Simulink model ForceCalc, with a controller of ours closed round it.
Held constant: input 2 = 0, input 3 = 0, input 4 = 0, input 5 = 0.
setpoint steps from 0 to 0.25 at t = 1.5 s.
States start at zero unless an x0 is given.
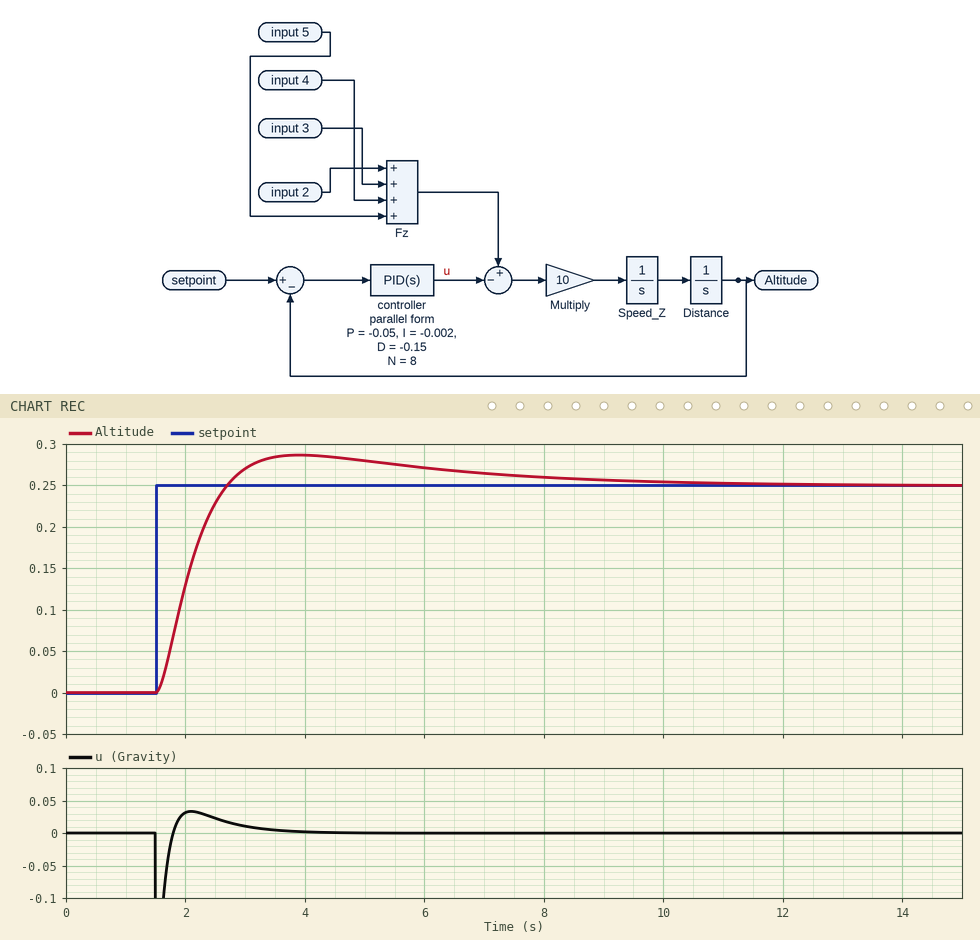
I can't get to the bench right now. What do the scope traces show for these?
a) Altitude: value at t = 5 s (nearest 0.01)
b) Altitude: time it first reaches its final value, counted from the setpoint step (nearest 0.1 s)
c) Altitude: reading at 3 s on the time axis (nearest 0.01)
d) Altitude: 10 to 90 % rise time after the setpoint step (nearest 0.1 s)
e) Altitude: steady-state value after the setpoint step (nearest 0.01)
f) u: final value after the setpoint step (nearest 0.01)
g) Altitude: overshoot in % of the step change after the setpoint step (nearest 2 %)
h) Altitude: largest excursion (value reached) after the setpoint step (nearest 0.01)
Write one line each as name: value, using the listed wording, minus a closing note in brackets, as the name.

Altitude: value at t = 5 s: 0.28
Altitude: time it first reaches its final value, counted from the setpoint step: 1.2 s
Altitude: reading at 3 s on the time axis: 0.27
Altitude: 10 to 90 % rise time after the setpoint step: 0.8 s
Altitude: steady-state value after the setpoint step: 0.25
u: final value after the setpoint step: 0.00
Altitude: overshoot in % of the step change after the setpoint step: 14 %
Altitude: largest excursion (value reached) after the setpoint step: 0.29
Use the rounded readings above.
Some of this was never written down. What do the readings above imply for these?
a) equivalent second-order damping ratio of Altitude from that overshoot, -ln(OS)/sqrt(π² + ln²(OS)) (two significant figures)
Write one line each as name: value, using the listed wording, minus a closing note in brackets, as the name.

equivalent second-order damping ratio of Altitude from that overshoot, -ln(OS)/sqrt(π² + ln²(OS)): 0.53
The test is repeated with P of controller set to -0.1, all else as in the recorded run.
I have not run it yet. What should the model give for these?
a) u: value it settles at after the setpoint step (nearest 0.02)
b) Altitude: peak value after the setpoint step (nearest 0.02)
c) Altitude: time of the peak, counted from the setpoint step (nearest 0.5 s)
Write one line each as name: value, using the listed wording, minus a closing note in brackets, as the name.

u: value it settles at after the setpoint step: 0.00
Altitude: peak value after the setpoint step: 0.30
Altitude: time of the peak, counted from the setpoint step: 2.0 s
